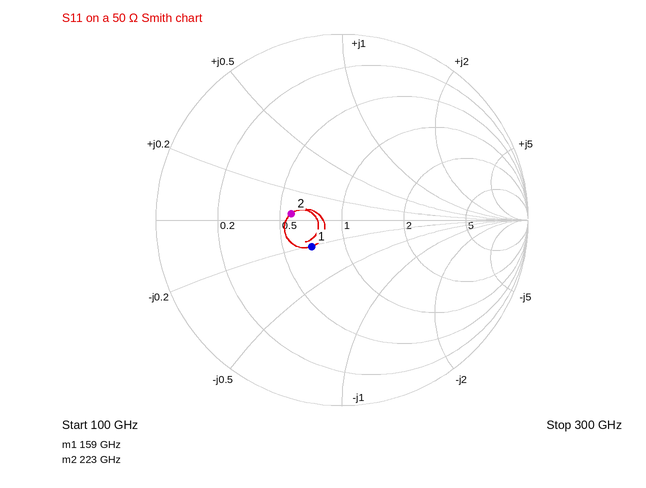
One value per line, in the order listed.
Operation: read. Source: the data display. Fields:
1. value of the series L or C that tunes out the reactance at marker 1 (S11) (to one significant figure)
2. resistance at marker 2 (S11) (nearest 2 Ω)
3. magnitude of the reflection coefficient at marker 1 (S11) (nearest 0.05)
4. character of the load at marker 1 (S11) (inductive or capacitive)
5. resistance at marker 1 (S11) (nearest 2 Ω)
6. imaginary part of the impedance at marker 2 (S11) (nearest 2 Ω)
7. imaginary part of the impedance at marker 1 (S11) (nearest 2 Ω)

10 pH
28 Ω
0.20
capacitive
34 Ω
+2 Ω
-10 Ω
